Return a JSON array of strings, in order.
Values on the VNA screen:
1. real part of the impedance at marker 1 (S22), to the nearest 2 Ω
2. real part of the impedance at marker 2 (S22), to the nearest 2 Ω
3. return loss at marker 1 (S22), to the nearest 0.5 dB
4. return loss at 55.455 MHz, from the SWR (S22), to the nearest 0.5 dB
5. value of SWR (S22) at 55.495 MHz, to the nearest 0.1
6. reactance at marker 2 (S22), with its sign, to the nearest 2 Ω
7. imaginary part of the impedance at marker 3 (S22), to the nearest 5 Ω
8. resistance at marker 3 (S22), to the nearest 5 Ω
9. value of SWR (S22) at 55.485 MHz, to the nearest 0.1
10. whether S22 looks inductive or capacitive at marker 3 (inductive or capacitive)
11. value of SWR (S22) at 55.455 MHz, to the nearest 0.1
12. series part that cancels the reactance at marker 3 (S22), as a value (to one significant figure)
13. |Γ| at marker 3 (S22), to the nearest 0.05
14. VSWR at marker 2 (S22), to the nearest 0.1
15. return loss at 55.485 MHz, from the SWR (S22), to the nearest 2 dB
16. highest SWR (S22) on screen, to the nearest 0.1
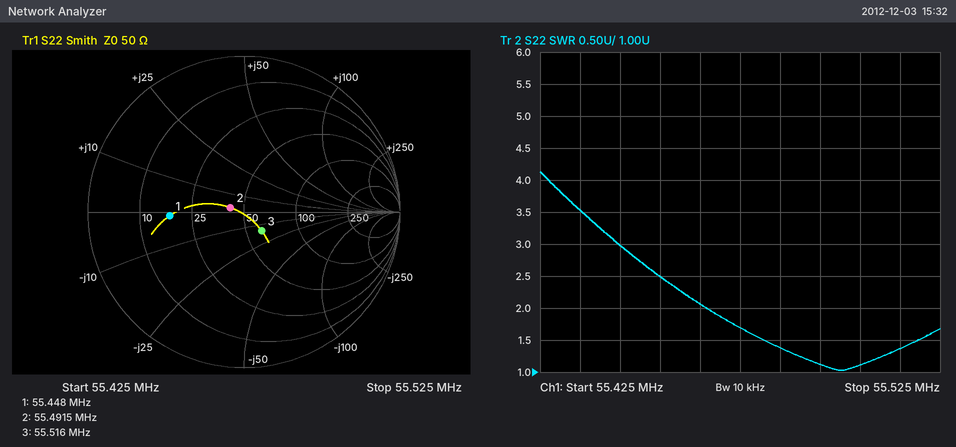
["18 Ω", "42 Ω", "6.5 dB", "7.5 dB", "1.1", "+2 Ω", "-15 Ω", "60 Ω", "1.4", "capacitive", "2.5", "40 nH", "0.15", "1.2", "16 dB", "4.1"]
